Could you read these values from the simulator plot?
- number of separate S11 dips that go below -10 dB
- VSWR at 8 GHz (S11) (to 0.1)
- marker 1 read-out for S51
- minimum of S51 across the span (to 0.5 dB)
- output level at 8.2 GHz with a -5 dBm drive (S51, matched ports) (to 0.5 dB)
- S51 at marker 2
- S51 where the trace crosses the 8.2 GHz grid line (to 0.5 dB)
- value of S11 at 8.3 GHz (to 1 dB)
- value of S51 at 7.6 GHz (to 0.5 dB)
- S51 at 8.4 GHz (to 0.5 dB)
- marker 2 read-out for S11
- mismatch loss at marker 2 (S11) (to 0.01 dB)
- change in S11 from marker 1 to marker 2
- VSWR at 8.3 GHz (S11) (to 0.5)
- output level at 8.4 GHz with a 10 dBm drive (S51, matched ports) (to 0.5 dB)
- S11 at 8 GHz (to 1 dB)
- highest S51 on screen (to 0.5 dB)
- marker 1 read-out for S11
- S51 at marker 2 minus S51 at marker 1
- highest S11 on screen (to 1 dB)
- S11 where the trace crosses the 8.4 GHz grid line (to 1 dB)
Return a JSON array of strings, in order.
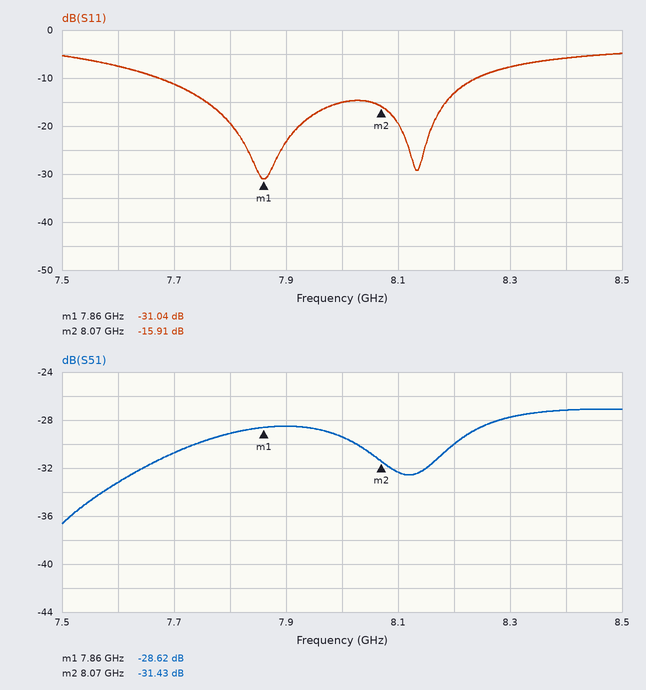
["2", "1.4", "-28.62 dB", "-36.5 dB", "-35.0 dBm", "-31.43 dB", "-30.0 dB", "-8 dB", "-33.0 dB", "-27.0 dB", "-15.91 dB", "0.11 dB", "15.13 dB", "2.5", "-17.0 dBm", "-15 dB", "-27.0 dB", "-31.04 dB", "-2.81 dB", "-5 dB", "-6 dB"]
